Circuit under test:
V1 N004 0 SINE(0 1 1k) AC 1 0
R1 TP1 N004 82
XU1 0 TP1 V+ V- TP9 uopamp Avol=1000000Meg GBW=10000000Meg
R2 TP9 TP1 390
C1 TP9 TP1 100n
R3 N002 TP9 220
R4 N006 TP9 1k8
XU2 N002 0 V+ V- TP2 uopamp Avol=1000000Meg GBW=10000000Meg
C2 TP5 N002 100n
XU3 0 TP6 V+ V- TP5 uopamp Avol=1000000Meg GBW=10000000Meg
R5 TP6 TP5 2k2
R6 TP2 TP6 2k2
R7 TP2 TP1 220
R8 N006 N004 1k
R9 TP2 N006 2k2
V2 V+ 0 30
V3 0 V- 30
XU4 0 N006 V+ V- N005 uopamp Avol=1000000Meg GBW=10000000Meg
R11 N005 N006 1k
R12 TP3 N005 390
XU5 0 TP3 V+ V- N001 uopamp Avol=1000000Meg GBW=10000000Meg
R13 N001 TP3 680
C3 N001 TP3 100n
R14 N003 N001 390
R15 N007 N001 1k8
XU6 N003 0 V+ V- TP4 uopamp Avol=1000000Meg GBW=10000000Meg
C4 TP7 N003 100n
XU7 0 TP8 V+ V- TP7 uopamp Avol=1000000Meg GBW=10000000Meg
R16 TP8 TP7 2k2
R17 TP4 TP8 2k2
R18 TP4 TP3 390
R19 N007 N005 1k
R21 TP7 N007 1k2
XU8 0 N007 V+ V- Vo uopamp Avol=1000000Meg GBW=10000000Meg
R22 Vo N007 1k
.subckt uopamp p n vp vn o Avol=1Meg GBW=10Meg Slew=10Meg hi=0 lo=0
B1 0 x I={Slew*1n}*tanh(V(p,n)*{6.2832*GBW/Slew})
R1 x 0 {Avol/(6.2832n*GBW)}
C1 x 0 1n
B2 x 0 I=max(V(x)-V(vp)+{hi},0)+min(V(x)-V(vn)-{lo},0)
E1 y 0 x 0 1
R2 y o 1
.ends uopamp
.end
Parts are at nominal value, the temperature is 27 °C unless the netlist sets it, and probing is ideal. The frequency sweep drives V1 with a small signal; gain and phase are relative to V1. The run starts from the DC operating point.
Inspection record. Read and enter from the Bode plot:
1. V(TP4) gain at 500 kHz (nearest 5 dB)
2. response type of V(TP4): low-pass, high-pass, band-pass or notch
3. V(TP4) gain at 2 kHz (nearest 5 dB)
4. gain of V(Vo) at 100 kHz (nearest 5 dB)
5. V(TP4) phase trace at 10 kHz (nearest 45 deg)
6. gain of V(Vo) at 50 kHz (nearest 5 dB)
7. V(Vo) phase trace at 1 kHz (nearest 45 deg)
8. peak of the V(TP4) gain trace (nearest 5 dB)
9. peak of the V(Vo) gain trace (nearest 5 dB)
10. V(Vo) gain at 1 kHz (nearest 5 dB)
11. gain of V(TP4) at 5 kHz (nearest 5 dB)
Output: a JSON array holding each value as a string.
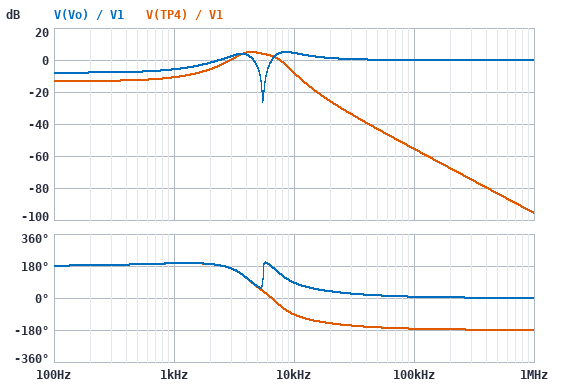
["-85 dB", "band-pass", "-5 dB", "0 dB", "-90 deg", "0 dB", "180 deg", "5 dB", "5 dB", "-5 dB", "5 dB"]
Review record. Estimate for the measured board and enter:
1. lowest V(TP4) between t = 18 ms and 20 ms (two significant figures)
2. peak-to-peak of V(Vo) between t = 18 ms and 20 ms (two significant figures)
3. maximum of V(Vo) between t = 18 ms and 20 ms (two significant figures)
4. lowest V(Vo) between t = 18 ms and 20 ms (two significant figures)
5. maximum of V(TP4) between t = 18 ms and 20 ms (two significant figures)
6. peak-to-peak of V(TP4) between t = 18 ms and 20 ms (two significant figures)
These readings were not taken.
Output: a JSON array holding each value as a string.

["-290 mV", "1.0 V", "510 mV", "-510 mV", "290 mV", "580 mV"]
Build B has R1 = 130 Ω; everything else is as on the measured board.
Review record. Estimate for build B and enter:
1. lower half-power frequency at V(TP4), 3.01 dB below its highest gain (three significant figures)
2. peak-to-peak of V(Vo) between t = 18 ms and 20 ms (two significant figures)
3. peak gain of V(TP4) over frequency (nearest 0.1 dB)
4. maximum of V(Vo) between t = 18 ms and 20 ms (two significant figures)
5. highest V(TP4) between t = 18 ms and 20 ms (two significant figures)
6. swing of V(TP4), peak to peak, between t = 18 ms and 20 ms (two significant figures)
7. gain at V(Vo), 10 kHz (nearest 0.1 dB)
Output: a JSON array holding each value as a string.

["3.88 kHz", "830 mV", "-3.2 dB", "410 mV", "230 mV", "470 mV", "1.4 dB"]
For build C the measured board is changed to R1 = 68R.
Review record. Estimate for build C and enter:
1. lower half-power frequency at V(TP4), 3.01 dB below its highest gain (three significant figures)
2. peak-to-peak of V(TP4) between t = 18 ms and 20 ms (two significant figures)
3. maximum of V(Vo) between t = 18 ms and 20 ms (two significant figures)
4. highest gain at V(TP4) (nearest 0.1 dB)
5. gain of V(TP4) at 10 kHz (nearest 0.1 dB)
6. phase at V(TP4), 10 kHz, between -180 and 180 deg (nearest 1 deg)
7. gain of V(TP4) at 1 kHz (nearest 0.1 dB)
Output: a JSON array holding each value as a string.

["3.22 kHz", "1.1 V", "980 mV", "7.8 dB", "-6.6 dB", "-88 deg", "-5.1 dB"]
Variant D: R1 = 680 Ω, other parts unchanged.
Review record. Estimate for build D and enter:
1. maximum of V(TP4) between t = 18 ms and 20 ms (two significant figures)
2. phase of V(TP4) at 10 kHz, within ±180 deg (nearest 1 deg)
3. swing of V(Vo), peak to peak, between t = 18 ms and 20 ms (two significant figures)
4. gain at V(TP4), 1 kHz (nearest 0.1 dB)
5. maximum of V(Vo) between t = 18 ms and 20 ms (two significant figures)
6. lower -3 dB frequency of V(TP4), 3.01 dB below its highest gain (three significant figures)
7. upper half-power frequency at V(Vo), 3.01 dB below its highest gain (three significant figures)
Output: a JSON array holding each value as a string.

["890 mV", "-150 deg", "3.2 V", "-1.0 dB", "1.6 V", "1.90 kHz", "4.00 kHz"]
